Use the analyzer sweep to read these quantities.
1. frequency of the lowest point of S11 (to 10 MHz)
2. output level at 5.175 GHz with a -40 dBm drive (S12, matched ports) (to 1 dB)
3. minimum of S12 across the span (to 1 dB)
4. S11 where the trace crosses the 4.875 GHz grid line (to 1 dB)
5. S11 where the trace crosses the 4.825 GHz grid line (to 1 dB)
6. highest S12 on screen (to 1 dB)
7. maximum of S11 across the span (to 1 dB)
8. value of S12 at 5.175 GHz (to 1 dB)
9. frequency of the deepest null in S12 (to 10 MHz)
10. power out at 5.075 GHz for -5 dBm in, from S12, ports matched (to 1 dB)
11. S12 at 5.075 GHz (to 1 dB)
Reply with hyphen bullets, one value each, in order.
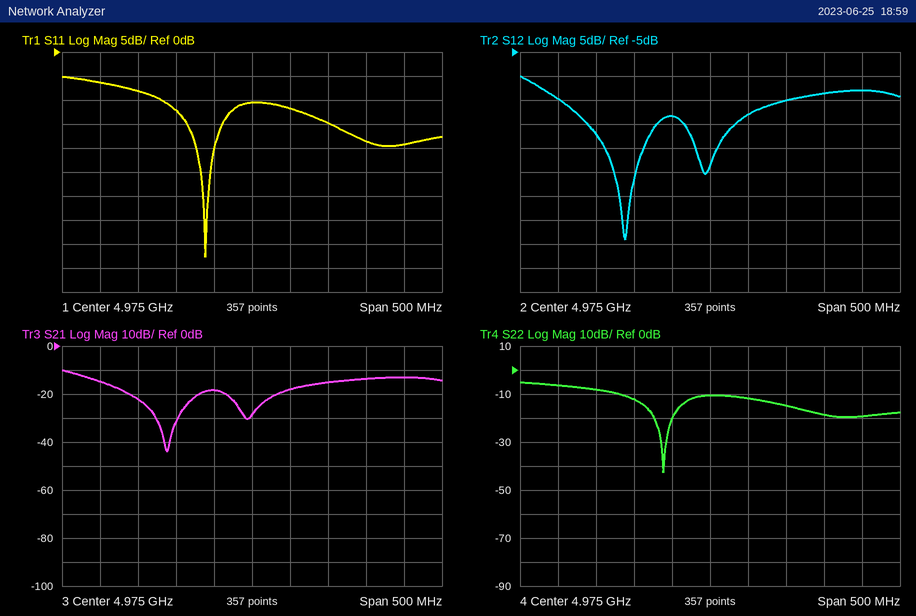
- 4.91 GHz
- -53 dBm
- -44 dB
- -12 dB
- -8 dB
- -10 dB
- -5 dB
- -13 dB
- 4.86 GHz
- -20 dBm
- -15 dB
